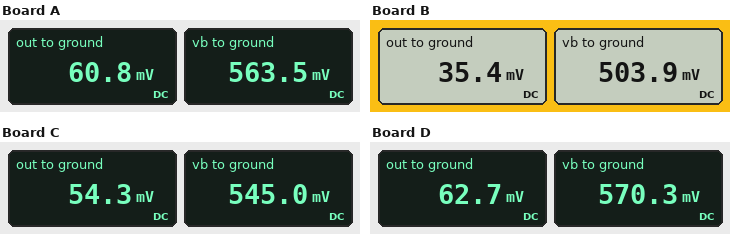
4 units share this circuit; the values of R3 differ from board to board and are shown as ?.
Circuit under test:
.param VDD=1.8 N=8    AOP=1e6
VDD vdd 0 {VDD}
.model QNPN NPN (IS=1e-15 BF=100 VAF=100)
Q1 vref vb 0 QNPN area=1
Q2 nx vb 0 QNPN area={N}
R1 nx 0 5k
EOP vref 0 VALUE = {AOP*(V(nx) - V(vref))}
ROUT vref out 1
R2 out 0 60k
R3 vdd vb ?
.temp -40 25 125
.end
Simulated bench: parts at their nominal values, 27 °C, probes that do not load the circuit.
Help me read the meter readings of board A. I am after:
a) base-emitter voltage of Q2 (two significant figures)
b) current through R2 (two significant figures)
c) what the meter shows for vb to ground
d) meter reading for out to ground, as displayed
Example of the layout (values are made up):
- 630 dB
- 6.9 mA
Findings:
- 560 mV
- 1.0 µA
- 563.5 mV
- 60.8 mV
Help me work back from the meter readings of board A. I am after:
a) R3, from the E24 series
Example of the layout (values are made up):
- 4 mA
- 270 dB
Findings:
- 68 kΩ
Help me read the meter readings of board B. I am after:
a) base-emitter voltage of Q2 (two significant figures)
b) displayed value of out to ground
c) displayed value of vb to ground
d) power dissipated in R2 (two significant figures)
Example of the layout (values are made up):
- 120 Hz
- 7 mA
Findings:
- 500 mV
- 35.4 mV
- 503.9 mV
- 21 nW
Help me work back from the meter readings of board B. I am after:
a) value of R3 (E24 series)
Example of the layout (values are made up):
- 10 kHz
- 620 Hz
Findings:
- 270 kΩ
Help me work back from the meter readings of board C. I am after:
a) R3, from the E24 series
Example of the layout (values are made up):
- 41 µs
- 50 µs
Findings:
- 110 kΩ
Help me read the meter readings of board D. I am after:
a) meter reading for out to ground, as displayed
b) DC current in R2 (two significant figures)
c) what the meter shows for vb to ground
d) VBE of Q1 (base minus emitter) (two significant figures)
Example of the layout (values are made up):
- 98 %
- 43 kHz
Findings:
- 62.7 mV
- 1.0 µA
- 570.3 mV
- 570 mV
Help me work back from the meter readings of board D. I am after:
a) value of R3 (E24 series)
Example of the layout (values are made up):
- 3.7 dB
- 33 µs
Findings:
- 56 kΩ
